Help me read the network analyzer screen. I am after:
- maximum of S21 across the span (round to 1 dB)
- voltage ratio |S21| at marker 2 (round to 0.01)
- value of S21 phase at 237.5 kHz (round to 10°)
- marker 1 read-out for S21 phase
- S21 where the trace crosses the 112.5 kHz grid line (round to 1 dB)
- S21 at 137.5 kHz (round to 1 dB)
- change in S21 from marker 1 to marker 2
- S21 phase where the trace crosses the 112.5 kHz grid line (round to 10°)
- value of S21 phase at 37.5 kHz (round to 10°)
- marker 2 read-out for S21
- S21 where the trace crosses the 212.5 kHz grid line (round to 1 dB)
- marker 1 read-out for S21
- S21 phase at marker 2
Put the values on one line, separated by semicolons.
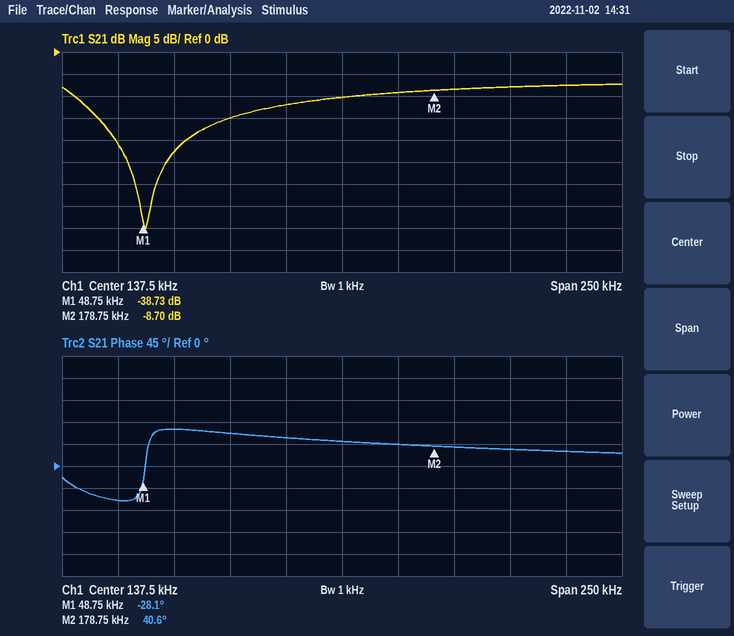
-7 dB; 0.37; 30°; -28.1°; -12 dB; -10 dB; 30.03 dB; 60°; -70°; -8.70 dB; -8 dB; -38.73 dB; 40.6°
